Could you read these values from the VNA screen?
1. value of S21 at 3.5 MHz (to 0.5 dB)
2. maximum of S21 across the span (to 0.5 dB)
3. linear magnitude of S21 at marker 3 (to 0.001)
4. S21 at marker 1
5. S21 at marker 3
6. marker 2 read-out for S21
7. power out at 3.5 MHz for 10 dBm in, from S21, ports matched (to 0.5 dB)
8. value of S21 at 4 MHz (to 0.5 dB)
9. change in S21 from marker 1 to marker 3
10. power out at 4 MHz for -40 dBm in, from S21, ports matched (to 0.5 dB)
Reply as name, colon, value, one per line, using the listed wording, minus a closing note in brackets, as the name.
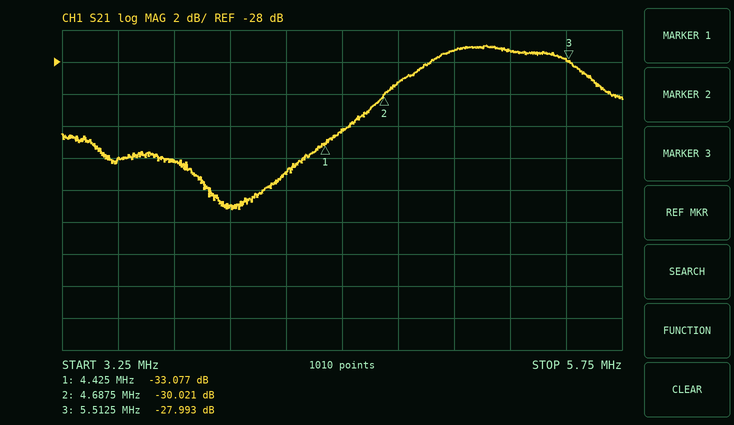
value of S21 at 3.5 MHz: -34.0 dB
maximum of S21 across the span: -27.0 dB
linear magnitude of S21 at marker 3: 0.040
S21 at marker 1: -33.077 dB
S21 at marker 3: -27.993 dB
marker 2 read-out for S21: -30.021 dB
power out at 3.5 MHz for 10 dBm in, from S21, ports matched: -24.0 dBm
value of S21 at 4 MHz: -37.0 dB
change in S21 from marker 1 to marker 3: 5.084 dB
power out at 4 MHz for -40 dBm in, from S21, ports matched: -77.0 dBm
